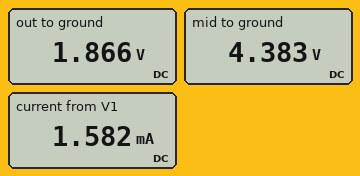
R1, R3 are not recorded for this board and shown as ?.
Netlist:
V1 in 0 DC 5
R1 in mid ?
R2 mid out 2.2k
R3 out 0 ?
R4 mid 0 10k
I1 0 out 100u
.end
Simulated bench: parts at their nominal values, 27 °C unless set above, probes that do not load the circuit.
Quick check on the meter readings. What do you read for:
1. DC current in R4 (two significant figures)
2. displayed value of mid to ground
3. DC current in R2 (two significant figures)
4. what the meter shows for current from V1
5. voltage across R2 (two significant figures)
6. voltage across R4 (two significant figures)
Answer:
440 µA
4.383 V
1.1 mA
1.582 mA
2.5 V
4.4 V
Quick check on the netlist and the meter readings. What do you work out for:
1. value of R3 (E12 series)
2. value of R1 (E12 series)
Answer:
1.5 kΩ
390 Ω
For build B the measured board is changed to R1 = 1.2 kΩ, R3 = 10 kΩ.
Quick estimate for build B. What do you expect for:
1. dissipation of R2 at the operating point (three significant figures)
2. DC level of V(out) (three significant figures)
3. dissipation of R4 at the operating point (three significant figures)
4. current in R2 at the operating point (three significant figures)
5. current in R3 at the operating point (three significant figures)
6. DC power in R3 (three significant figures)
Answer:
150 µW
3.61 V
1.75 mW
261 µA
361 µA
1.30 mW
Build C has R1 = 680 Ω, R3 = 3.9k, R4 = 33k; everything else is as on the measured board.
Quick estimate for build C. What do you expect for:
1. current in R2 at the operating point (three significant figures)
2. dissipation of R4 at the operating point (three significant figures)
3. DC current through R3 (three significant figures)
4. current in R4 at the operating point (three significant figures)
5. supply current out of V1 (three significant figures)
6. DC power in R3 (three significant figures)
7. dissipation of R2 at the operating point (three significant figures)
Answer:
666 µA
601 µW
766 µA
135 µA
801 µA
2.29 mW
977 µW
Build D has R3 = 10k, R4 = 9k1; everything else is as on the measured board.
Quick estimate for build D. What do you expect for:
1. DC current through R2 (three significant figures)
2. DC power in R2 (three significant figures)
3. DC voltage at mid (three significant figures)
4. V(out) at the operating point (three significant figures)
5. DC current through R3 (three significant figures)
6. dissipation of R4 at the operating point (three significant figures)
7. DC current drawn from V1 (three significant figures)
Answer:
302 µA
200 µW
4.68 V
4.02 V
402 µA
2.41 mW
816 µA
